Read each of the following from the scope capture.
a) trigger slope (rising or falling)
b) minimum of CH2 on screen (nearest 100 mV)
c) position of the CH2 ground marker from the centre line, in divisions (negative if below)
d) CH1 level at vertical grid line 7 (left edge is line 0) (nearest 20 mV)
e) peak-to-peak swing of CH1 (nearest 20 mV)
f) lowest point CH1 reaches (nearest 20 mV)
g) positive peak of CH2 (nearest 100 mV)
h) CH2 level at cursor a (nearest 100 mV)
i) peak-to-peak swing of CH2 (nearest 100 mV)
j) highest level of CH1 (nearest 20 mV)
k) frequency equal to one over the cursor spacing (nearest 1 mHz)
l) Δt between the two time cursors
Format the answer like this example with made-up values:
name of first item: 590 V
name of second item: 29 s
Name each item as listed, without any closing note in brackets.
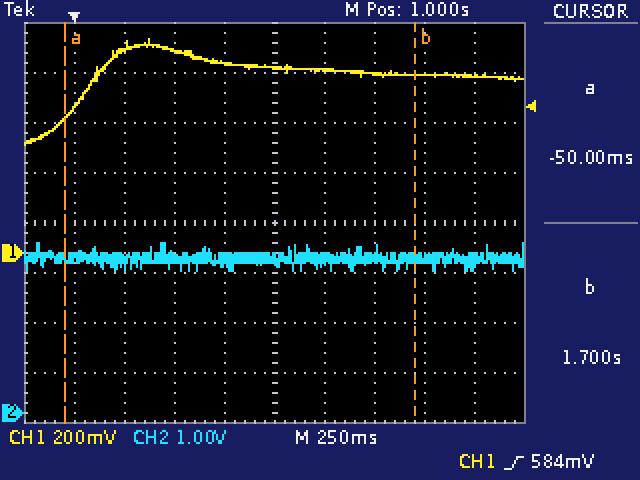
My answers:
trigger slope: rising
minimum of CH2 on screen: 2.8 V
position of the CH2 ground marker from the centre line, in divisions: -3.8 div
CH1 level at vertical grid line 7 (left edge is line 0): 720 mV
peak-to-peak swing of CH1: 420 mV
lowest point CH1 reaches: 440 mV
positive peak of CH2: 3.4 V
CH2 level at cursor a: 3.1 V
peak-to-peak swing of CH2: 600 mV
highest level of CH1: 860 mV
frequency equal to one over the cursor spacing: 571 mHz
Δt between the two time cursors: 1.750 s
